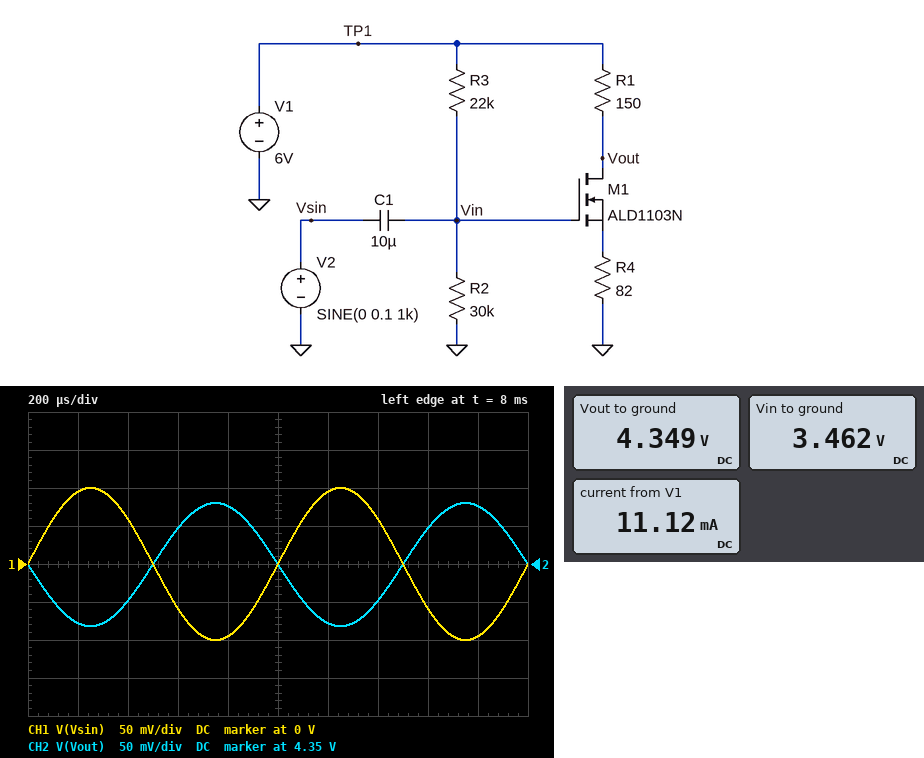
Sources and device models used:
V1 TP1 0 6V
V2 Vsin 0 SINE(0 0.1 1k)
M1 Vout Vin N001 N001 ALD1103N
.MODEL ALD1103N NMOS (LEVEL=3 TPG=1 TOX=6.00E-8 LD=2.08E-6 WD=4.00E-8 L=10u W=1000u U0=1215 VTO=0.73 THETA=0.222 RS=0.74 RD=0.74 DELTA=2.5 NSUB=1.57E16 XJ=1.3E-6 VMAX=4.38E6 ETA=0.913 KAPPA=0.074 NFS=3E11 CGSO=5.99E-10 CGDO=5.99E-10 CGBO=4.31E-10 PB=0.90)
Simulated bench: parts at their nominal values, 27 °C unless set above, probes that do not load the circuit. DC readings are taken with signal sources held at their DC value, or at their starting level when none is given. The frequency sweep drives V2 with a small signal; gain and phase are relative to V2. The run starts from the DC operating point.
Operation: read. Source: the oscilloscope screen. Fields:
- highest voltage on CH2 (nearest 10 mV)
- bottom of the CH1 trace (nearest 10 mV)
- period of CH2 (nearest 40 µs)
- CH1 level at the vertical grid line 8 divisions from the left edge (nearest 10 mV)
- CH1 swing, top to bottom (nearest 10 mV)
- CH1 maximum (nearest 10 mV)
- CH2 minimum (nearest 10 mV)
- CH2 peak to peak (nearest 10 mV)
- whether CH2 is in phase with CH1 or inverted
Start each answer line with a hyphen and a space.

- 4.43 V
- -100 mV
- 1.00 ms
- -60 mV
- 200 mV
- 100 mV
- 4.27 V
- 160 mV
- inverted
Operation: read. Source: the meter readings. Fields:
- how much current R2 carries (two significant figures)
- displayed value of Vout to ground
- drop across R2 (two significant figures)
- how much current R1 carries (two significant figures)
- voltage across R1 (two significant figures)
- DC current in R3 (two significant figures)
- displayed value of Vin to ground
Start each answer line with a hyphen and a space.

- 120 µA
- 4.349 V
- 3.5 V
- 11 mA
- 1.7 V
- 120 µA
- 3.462 V
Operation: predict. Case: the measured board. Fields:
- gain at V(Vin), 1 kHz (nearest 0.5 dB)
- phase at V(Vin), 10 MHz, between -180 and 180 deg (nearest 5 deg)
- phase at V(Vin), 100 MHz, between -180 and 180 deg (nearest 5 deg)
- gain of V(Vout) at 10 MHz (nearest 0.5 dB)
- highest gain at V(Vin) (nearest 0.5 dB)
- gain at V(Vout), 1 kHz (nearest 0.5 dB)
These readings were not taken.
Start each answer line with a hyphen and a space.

- 0 dB
- 0 deg
- 0 deg
- -2.0 dB
- 0 dB
- -2.0 dB
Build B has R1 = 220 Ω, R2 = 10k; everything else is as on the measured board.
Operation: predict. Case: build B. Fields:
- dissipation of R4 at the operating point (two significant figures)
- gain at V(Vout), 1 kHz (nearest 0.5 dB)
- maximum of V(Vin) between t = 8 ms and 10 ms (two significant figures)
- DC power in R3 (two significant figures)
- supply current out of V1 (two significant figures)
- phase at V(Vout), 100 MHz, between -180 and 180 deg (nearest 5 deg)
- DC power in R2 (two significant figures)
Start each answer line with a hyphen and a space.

- 880 µW
- -1.0 dB
- 2.0 V
- 770 µW
- 3.5 mA
- 165 deg
- 350 µW
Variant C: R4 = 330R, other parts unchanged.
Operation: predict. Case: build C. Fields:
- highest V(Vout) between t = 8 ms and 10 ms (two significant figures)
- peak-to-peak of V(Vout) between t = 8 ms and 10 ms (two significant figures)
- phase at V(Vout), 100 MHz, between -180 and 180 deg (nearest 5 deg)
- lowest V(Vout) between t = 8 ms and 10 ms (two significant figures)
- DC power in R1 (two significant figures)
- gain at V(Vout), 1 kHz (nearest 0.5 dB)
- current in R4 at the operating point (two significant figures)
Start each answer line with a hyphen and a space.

- 5.3 V
- 64 mV
- 155 deg
- 5.2 V
- 3.6 mW
- -10.0 dB
- 4.9 mA
